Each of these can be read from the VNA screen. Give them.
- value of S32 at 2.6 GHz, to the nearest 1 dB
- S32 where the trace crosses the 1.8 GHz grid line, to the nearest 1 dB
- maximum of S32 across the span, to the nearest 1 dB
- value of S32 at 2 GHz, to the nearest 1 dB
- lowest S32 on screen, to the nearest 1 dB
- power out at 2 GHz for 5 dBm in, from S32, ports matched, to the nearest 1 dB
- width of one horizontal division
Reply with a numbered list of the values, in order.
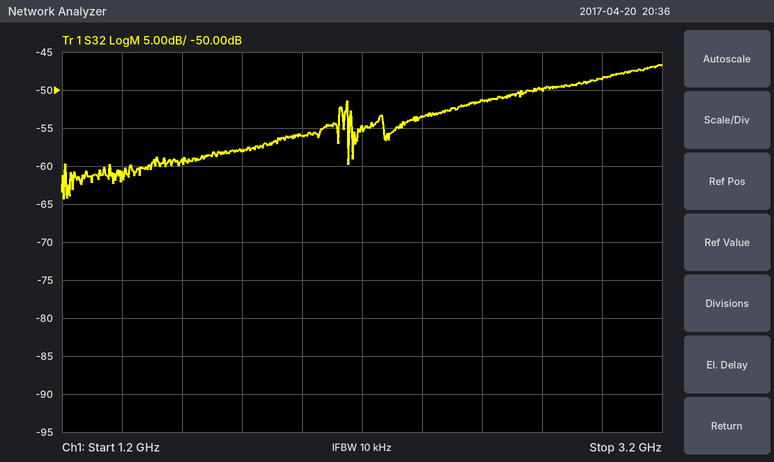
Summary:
1. -51 dB
2. -58 dB
3. -47 dB
4. -56 dB
5. -64 dB
6. -51 dBm
7. 200 MHz
